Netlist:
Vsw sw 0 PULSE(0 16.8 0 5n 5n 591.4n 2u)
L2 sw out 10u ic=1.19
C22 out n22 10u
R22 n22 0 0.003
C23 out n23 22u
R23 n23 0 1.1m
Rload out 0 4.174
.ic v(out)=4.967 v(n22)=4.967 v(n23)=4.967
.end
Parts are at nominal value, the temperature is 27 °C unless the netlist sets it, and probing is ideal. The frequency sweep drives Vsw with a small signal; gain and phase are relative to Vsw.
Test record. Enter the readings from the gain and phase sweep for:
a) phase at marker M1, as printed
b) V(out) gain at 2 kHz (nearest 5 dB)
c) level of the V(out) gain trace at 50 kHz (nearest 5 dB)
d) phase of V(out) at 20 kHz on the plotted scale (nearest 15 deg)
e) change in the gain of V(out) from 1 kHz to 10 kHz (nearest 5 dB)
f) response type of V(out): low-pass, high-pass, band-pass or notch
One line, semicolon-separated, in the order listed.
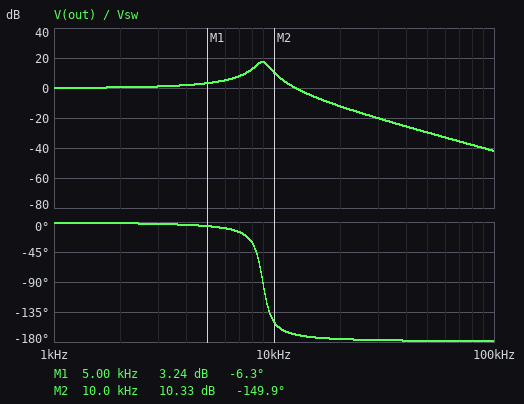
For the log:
-6.3 deg; 0 dB; -30 dB; -180 deg; 10 dB; low-pass
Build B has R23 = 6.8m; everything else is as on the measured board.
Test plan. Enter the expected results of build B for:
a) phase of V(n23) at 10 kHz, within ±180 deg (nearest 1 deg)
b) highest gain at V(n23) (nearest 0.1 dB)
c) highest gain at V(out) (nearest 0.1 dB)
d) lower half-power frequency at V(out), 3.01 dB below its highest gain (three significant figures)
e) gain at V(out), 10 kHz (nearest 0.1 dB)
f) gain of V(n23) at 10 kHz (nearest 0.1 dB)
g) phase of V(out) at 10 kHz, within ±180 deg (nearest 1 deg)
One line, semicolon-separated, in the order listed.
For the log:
-59 deg; -24.5 dB; 17.1 dB; 8.20 kHz; 10.2 dB; -30.3 dB; -149 deg
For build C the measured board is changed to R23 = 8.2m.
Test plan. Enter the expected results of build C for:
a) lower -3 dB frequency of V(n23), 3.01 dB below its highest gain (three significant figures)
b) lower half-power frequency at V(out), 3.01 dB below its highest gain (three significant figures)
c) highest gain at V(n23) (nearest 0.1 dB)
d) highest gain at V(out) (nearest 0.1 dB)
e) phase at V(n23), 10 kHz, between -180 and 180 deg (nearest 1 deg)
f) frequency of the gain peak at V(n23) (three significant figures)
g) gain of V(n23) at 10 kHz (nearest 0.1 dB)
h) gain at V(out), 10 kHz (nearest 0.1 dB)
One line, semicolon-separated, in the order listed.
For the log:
8.29 kHz; 8.19 kHz; -22.9 dB; 17.0 dB; -59 deg; 8.89 kHz; -28.7 dB; 10.2 dB
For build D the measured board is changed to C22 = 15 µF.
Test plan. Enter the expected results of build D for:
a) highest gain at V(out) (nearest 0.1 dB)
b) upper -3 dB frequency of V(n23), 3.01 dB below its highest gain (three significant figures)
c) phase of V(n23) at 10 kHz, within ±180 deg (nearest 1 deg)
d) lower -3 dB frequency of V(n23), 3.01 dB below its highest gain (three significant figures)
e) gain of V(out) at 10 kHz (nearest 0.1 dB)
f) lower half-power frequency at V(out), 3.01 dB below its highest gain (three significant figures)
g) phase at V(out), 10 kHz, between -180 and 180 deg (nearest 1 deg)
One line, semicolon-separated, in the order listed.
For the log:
18.0 dB; 8.81 kHz; -72 deg; 7.77 kHz; 6.3 dB; 7.70 kHz; -162 deg
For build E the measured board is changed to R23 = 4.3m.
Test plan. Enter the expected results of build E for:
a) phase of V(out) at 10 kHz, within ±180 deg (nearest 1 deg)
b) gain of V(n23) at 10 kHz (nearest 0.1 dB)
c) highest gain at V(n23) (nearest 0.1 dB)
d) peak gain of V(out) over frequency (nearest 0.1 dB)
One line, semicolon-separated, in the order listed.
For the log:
-149 deg; -34.2 dB; -28.3 dB; 17.2 dB
